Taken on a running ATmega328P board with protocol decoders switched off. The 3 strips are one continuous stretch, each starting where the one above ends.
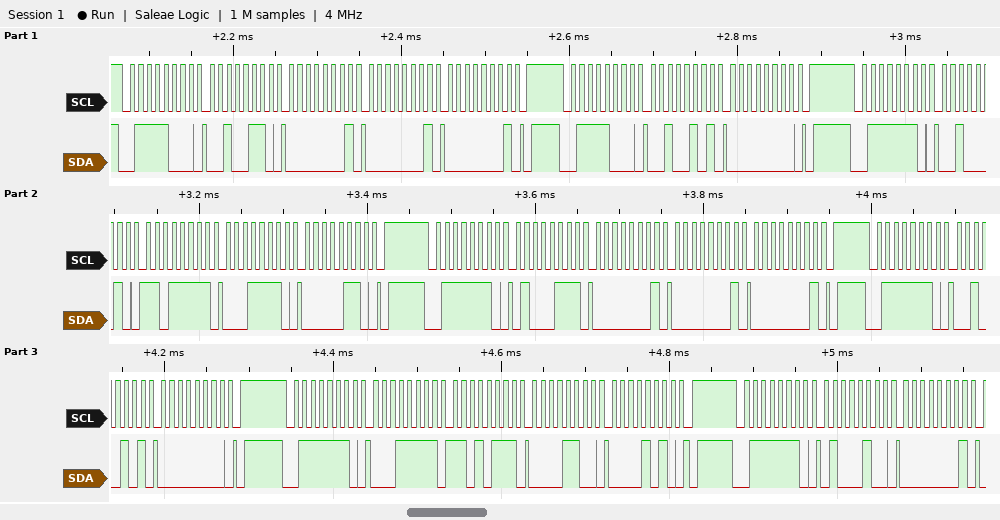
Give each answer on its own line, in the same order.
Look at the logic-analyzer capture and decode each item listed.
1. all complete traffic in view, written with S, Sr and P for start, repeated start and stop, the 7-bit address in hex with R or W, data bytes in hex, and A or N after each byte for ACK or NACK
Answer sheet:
S 3CW A 26 A 01 A 01 A 01 A P S 3CW A 25 A 00 A P S 3FW A 22 A DF A 1E A 06 A P S 3FW A 47 A 01 A 01 A 01 A P S 3FW A 25 A 00 A P S 3FW A 1F A D7 A 0C A 0A A P S 3FW A 44 A 01 A
